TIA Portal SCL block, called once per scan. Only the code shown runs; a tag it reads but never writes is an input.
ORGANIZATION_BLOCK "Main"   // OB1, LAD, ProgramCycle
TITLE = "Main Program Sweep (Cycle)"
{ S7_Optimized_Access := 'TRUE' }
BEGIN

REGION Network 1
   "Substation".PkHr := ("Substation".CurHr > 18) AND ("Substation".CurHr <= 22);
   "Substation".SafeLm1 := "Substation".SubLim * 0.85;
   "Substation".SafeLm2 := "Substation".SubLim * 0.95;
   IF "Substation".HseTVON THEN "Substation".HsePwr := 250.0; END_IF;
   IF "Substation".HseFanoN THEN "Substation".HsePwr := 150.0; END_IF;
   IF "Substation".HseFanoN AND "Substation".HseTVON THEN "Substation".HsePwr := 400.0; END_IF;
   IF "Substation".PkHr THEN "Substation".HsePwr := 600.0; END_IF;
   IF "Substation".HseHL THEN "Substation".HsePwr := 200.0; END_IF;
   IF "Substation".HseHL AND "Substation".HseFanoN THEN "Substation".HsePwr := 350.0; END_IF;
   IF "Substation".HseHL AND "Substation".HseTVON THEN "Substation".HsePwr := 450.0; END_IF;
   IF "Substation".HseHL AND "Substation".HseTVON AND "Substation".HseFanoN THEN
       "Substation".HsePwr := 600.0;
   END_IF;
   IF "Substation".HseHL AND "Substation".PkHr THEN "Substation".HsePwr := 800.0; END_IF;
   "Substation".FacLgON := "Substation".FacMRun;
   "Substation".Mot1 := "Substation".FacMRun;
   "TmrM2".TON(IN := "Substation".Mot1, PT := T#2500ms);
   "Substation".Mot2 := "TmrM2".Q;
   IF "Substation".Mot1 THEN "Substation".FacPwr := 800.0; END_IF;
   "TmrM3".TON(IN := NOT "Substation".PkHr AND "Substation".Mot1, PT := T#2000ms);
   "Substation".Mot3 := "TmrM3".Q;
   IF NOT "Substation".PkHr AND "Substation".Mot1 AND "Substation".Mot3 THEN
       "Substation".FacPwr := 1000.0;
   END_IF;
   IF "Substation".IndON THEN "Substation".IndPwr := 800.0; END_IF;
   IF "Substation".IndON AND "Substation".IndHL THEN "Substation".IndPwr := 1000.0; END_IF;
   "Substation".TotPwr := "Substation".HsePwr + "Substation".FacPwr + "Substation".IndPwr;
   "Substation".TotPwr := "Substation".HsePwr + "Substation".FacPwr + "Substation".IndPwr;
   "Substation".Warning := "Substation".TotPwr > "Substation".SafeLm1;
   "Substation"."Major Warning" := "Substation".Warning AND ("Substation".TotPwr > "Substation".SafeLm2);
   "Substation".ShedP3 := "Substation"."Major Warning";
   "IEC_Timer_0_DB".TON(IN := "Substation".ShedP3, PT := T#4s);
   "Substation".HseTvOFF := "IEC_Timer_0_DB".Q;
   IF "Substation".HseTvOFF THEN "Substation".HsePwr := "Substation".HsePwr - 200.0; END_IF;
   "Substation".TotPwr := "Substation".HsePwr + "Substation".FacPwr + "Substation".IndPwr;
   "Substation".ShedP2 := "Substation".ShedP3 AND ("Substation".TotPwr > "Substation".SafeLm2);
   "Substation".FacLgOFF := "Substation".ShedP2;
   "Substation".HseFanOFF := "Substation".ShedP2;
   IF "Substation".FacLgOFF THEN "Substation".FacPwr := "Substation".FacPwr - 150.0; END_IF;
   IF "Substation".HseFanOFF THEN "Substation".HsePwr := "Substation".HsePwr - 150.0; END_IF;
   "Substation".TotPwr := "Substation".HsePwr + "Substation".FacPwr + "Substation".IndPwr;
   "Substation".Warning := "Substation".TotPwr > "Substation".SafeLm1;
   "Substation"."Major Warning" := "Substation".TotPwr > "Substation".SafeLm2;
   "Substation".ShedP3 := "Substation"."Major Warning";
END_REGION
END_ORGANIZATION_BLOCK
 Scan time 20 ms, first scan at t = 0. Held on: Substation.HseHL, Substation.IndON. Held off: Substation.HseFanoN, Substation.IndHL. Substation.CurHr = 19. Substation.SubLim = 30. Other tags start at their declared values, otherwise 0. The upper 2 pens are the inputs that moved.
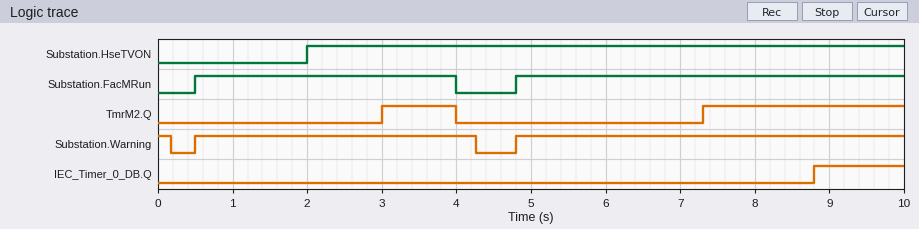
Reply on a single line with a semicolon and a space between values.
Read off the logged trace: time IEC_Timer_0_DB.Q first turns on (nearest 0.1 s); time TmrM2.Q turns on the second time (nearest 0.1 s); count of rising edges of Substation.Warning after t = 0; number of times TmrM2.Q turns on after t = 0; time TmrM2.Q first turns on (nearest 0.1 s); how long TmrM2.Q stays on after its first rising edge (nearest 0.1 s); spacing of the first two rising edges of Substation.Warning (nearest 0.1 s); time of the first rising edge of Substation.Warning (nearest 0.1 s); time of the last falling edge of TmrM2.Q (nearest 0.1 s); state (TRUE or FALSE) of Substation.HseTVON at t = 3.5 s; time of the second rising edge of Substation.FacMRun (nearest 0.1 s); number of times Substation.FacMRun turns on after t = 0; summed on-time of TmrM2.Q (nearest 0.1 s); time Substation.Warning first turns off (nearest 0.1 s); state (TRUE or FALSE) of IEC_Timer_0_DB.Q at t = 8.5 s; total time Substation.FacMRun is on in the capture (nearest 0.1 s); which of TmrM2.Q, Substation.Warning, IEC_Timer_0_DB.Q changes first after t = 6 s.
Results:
8.8 s; 7.3 s; 2; 2; 3.0 s; 1.0 s; 4.3 s; 0.5 s; 4.0 s; TRUE; 4.8 s; 2; 3.7 s; 0.2 s; FALSE; 8.7 s; TmrM2.Q
